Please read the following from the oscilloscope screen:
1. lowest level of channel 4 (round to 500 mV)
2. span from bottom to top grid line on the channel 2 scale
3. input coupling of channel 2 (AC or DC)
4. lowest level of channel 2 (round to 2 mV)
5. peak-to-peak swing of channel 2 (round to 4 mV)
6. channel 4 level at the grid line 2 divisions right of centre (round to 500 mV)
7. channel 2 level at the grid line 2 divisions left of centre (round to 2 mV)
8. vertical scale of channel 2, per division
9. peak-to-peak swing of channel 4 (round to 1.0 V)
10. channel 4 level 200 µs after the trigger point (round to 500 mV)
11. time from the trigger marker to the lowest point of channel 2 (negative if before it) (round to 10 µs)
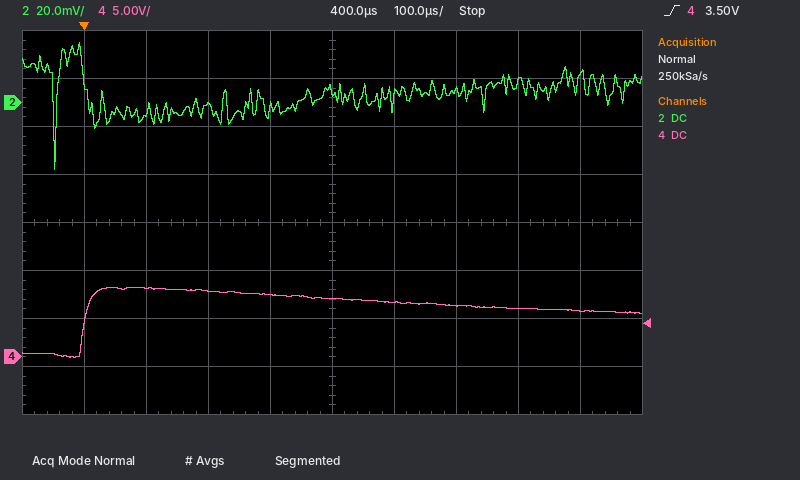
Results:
0.0 V
160 mV
DC
-28 mV
52 mV
5.5 V
0 mV
20 mV
7.0 V
7.0 V
-50 µs
